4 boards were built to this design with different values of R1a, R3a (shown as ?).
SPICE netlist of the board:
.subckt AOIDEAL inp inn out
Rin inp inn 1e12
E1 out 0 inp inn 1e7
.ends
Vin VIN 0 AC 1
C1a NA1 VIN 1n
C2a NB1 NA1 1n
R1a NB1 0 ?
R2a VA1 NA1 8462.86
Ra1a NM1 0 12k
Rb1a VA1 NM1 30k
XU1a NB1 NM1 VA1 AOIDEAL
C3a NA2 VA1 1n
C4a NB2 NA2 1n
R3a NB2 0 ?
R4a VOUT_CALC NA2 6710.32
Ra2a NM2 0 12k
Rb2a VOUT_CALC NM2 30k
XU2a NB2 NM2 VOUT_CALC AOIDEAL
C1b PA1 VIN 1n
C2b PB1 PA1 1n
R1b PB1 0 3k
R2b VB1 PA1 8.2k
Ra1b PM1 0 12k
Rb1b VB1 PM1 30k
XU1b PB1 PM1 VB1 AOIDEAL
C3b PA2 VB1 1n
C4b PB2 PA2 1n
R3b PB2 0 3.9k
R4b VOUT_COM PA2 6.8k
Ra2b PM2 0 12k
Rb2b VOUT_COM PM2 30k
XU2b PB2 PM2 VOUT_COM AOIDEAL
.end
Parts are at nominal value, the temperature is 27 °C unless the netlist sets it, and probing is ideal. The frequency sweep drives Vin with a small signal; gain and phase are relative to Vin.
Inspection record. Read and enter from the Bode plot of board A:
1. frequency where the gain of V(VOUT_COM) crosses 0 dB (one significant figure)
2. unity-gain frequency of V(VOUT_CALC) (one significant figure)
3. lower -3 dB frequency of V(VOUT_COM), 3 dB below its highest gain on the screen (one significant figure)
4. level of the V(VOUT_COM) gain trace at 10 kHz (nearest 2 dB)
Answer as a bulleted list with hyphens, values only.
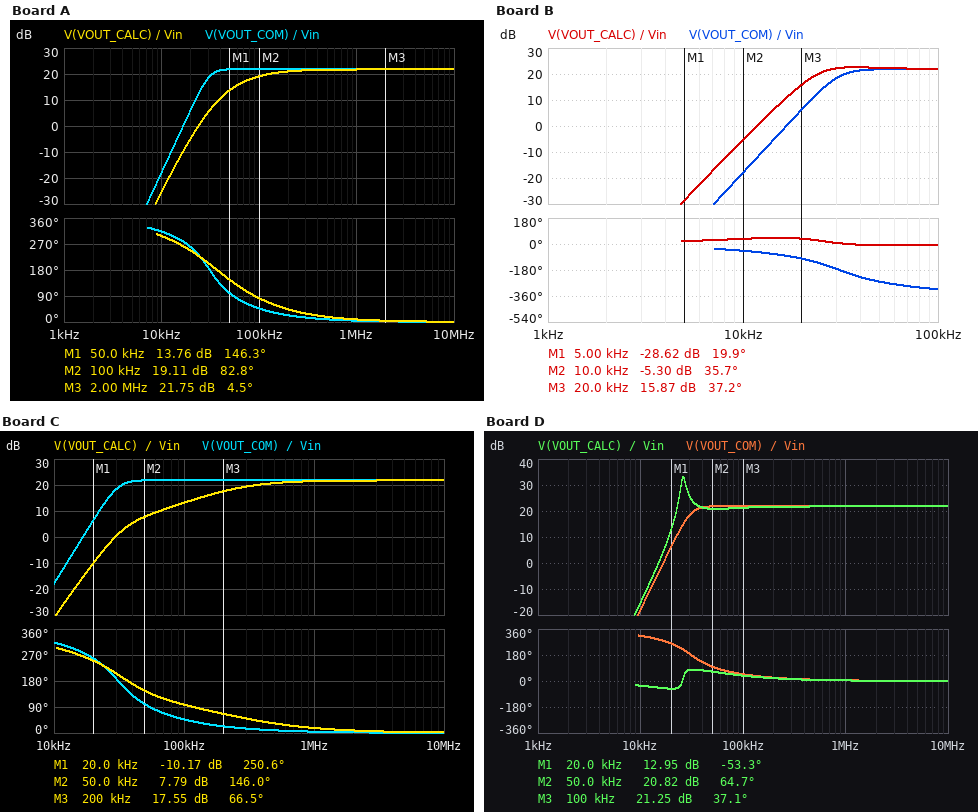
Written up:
- 20 kHz
- 20 kHz
- 30 kHz
- -18 dB
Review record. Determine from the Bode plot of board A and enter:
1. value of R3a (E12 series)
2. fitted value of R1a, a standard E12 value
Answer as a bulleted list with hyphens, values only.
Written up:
- 2.7 kΩ
- 2.2 kΩ
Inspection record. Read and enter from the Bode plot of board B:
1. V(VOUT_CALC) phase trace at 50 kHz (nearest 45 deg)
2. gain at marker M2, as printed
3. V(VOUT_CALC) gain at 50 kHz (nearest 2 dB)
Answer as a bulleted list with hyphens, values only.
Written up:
- 0 deg
- -5.30 dB
- 22 dB
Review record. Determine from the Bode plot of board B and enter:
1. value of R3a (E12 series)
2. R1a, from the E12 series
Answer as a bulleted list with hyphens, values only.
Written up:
- 12 kΩ
- 4.7 kΩ
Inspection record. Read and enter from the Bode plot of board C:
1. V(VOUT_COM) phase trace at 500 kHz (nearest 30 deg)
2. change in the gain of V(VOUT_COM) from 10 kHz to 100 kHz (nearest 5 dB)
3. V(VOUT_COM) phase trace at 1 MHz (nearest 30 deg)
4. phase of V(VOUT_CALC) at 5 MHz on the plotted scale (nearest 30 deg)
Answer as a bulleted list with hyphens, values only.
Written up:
- 0 deg
- 40 dB
- 0 deg
- 0 deg
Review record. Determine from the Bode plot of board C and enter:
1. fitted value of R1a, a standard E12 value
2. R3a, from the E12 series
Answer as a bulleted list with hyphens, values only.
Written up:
- 1 kΩ
- 3.3 kΩ
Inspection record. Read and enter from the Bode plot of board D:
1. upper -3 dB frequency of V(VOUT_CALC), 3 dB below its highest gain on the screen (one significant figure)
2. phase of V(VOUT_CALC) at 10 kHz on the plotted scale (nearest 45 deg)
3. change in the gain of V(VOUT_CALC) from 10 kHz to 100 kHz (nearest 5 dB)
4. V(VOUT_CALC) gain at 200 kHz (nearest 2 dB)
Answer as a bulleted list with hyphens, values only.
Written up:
- 30 kHz
- -45 deg
- 35 dB
- 22 dB
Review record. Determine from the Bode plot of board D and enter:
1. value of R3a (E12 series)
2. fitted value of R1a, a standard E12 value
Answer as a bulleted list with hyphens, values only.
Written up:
- 5.6 kΩ
- 2.7 kΩ
